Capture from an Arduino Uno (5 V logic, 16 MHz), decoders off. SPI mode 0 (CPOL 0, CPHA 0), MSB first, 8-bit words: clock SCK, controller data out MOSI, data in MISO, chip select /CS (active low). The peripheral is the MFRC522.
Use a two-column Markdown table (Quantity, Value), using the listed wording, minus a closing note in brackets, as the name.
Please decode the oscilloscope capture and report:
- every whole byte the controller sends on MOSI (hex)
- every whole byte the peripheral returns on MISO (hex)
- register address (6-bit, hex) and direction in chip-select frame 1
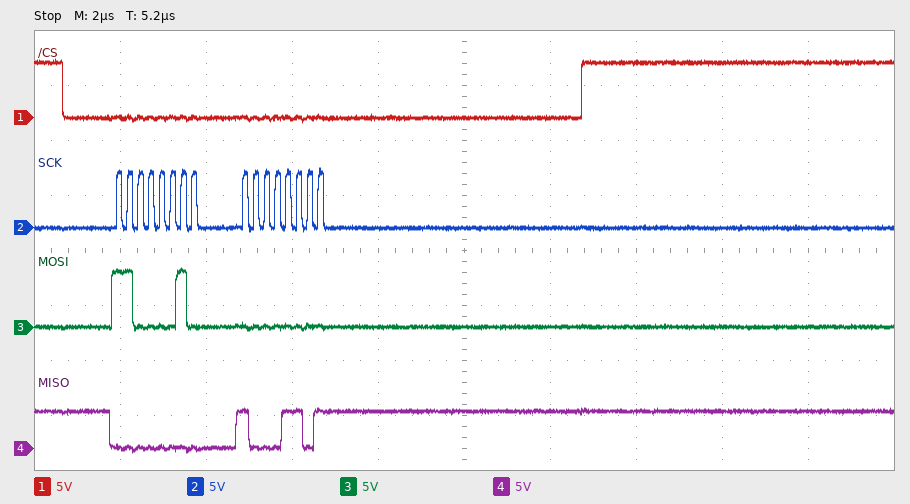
| Quantity | Value |
|---|---|
| every whole byte the controller sends on MOSI | C2 00 |
| every whole byte the peripheral returns on MISO | 00 8D |
| register address (6-bit, hex) and direction in chip-select frame 1 | 0x21 read |
